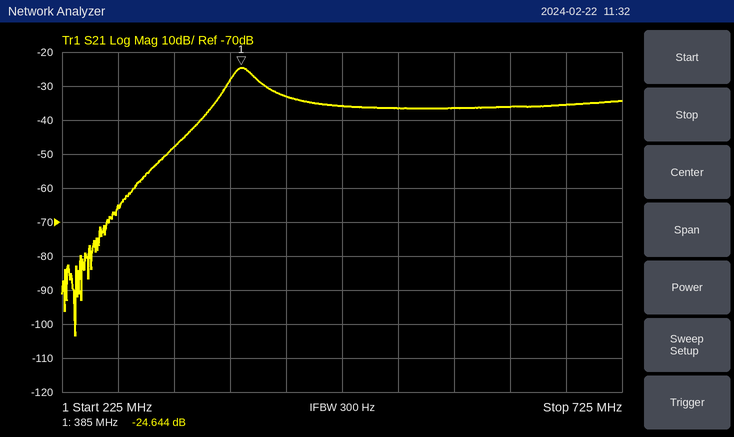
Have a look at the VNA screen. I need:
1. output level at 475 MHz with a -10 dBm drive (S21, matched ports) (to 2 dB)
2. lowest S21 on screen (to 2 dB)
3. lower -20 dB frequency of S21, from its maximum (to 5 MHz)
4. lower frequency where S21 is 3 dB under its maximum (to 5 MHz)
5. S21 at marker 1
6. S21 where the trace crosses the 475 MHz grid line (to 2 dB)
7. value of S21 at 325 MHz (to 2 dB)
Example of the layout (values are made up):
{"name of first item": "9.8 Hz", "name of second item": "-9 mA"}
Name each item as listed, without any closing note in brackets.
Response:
{"output level at 475 MHz with a -10 dBm drive (S21, matched ports)": "-46 dBm", "lowest S21 on screen": "-104 dB", "lower -20 dB frequency of S21, from its maximum": "335 MHz", "lower frequency where S21 is 3 dB under its maximum": "375 MHz", "S21 at marker 1": "-24.644 dB", "S21 where the trace crosses the 475 MHz grid line": "-36 dB", "value of S21 at 325 MHz": "-48 dB"}
